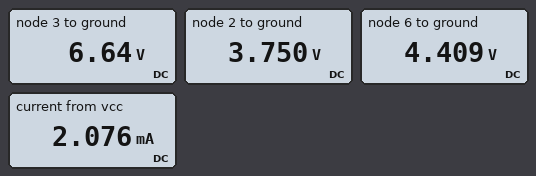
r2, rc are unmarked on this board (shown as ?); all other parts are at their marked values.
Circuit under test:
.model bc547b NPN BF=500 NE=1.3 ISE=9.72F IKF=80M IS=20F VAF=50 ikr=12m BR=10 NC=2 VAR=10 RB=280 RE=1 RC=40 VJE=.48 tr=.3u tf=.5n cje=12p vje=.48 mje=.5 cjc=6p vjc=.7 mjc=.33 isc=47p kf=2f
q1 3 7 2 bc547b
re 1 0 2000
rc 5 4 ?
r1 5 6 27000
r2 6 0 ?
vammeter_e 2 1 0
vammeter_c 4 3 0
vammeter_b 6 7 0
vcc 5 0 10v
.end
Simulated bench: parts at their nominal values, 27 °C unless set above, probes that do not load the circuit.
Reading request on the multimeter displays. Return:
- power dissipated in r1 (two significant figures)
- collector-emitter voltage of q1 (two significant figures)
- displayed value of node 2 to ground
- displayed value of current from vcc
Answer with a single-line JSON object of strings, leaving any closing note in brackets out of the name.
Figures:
{"power dissipated in r1": "1.2 mW", "collector-emitter voltage of q1": "2.9 V", "displayed value of node 2 to ground": "3.750 V", "displayed value of current from vcc": "2.076 mA"}
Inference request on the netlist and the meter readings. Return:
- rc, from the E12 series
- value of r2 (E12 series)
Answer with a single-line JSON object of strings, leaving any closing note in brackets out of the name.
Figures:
{"rc, from the E12 series": "1.8 kΩ", "value of r2": "22 kΩ"}
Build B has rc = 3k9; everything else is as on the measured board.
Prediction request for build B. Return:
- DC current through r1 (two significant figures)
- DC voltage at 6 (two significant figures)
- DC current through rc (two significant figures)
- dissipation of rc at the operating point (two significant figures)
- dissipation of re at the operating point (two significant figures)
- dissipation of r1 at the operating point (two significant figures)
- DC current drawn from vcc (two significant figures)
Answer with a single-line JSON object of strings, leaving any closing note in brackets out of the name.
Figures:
{"DC current through r1": "220 µA", "DC voltage at 6": "4.1 V", "DC current through rc": "1.7 mA", "dissipation of rc at the operating point": "11 mW", "dissipation of re at the operating point": "5.8 mW", "dissipation of r1 at the operating point": "1.3 mW", "DC current drawn from vcc": "1.9 mA"}
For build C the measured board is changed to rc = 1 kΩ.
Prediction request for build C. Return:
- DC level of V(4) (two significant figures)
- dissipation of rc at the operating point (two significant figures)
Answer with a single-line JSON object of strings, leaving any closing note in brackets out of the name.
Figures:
{"DC level of V(4)": "8.1 V", "dissipation of rc at the operating point": "3.5 mW"}
